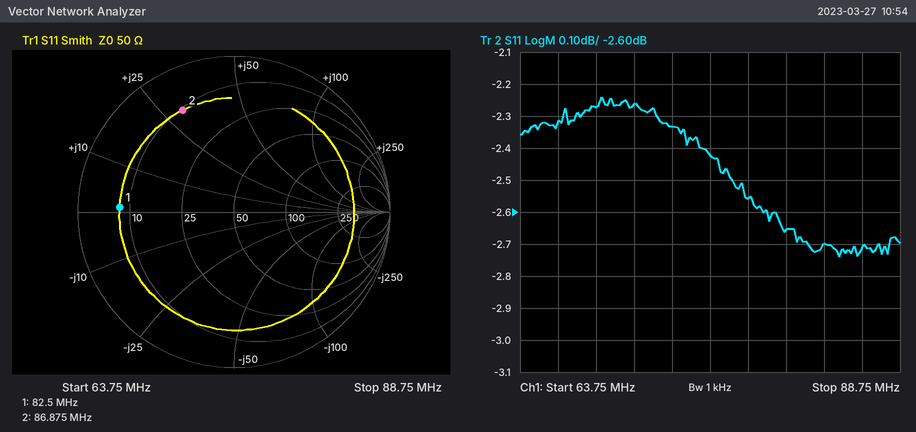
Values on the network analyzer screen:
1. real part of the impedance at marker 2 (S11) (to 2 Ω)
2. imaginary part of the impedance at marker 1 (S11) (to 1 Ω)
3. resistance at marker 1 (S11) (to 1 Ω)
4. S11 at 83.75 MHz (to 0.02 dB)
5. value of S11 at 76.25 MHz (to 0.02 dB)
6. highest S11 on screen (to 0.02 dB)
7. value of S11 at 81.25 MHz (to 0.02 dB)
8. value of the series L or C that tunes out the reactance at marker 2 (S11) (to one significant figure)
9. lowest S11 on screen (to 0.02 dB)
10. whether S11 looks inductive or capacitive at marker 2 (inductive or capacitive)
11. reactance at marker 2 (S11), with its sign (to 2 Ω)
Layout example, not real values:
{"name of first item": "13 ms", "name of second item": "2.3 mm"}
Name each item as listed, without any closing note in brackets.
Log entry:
{"real part of the impedance at marker 2 (S11)": "10 Ω", "imaginary part of the impedance at marker 1 (S11)": "+1 Ω", "resistance at marker 1 (S11)": "8 Ω", "S11 at 83.75 MHz": "-2.70 dB", "value of S11 at 76.25 MHz": "-2.42 dB", "highest S11 on screen": "-2.24 dB", "value of S11 at 81.25 MHz": "-2.66 dB", "value of the series L or C that tunes out the reactance at marker 2 (S11)": "60 pF", "lowest S11 on screen": "-2.74 dB", "whether S11 looks inductive or capacitive at marker 2": "inductive", "reactance at marker 2 (S11), with its sign": "+30 Ω"}
